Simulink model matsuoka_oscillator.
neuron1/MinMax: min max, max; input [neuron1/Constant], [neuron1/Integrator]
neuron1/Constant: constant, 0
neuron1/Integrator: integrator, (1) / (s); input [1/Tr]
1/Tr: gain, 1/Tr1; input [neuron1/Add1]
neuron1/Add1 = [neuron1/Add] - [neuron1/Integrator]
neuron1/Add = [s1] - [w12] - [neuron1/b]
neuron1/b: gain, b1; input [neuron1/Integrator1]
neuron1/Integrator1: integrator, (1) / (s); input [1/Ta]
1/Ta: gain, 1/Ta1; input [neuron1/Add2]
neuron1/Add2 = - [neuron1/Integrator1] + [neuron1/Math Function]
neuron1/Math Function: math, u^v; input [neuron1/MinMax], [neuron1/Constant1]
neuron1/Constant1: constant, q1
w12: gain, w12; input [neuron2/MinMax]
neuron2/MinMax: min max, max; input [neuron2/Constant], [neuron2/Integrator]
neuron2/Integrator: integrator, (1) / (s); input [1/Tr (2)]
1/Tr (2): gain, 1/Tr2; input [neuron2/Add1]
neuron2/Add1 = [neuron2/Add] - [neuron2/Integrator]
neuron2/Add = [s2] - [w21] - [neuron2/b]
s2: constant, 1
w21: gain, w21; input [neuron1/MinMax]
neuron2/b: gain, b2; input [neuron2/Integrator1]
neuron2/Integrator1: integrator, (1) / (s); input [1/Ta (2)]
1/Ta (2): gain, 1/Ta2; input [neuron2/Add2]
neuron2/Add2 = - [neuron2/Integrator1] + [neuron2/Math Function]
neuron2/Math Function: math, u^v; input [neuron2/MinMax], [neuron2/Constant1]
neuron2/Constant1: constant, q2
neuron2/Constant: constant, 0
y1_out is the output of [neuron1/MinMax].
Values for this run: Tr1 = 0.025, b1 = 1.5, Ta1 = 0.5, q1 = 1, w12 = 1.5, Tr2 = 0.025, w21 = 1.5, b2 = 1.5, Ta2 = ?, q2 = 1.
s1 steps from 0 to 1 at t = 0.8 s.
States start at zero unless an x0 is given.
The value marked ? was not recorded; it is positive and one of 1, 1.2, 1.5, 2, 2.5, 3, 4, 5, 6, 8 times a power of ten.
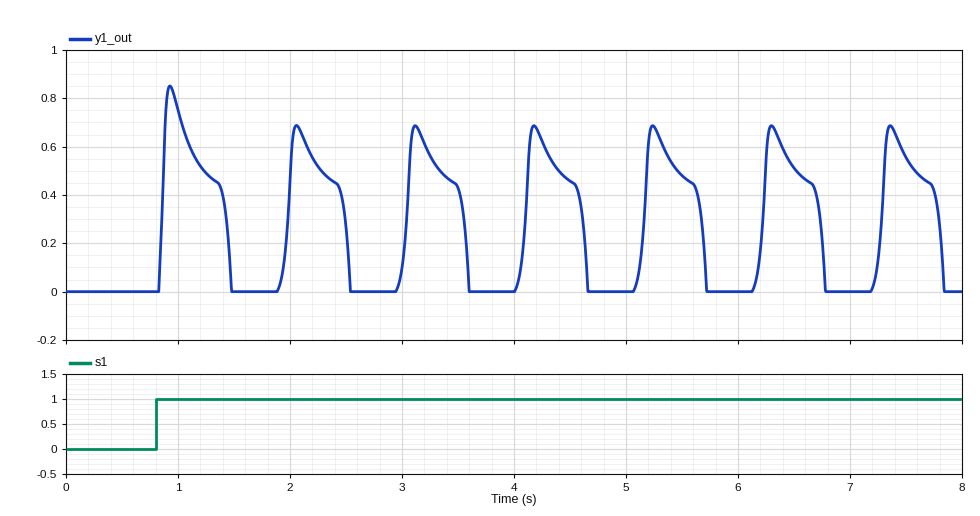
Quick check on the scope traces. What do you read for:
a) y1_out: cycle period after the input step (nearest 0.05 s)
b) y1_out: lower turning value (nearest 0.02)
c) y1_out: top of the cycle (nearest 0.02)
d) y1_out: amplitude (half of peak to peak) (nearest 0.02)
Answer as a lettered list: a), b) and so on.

a) 1.05 s
b) 0.00
c) 0.68
d) 0.34
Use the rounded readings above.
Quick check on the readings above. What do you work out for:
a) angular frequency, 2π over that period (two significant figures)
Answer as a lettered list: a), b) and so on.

a) 6.0 rad/s
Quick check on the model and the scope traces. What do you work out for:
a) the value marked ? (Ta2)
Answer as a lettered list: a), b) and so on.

a) 0.8
